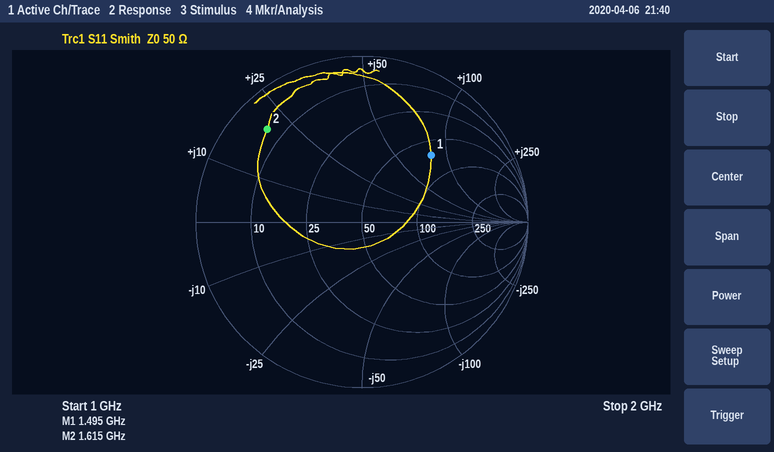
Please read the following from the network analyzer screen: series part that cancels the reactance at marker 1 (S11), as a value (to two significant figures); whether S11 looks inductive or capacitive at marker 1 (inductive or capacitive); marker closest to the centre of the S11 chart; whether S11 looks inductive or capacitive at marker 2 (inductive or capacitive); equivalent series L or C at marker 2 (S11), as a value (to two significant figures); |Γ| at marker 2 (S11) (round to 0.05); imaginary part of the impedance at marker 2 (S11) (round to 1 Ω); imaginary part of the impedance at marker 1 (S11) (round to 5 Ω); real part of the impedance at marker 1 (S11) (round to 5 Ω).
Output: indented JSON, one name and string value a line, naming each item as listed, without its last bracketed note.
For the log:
{
  "series part that cancels the reactance at marker 1 (S11), as a value": "1.3 pF",
  "whether S11 looks inductive or capacitive at marker 1": "inductive",
  "marker closest to the centre of the S11 chart": "marker 1",
  "whether S11 looks inductive or capacitive at marker 2": "inductive",
  "equivalent series L or C at marker 2 (S11), as a value": "2.0 nH",
  "|Γ| at marker 2 (S11)": "0.80",
  "imaginary part of the impedance at marker 2 (S11)": "+20 Ω",
  "imaginary part of the impedance at marker 1 (S11)": "+80 Ω",
  "real part of the impedance at marker 1 (S11)": "65 Ω"
}
